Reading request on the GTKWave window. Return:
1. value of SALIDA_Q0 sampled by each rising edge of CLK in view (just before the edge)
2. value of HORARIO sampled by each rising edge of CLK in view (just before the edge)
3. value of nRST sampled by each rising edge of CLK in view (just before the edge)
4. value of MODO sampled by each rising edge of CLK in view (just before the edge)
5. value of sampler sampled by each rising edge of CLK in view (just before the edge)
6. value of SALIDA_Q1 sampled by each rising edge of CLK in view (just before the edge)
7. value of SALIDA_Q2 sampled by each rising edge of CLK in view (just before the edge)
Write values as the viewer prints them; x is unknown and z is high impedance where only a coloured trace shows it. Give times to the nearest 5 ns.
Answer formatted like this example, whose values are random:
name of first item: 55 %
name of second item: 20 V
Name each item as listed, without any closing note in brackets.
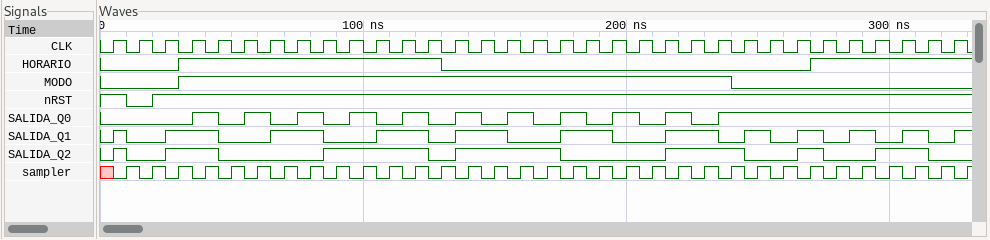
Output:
value of SALIDA_Q0 sampled by each rising edge of CLK in view: 0 0 0 0 1 0 1 0 1 0 1 0 1 0 1 0 1 0 1 0 1 0 1 0 1 1 1 1 1 1 1 1 1
value of HORARIO sampled by each rising edge of CLK in view: 0 0 0 1 1 1 1 1 1 1 1 1 1 0 0 0 0 0 0 0 0 0 0 0 0 0 0 1 1 1 1 1 1
value of nRST sampled by each rising edge of CLK in view: 1 0 1 1 1 1 1 1 1 1 1 1 1 1 1 1 1 1 1 1 1 1 1 1 1 1 1 1 1 1 1 1 1
value of MODO sampled by each rising edge of CLK in view: 0 0 0 1 1 1 1 1 1 1 1 1 1 1 1 1 1 1 1 1 1 1 1 1 0 0 0 0 0 0 0 0 0
value of sampler sampled by each rising edge of CLK in view: x 1 1 1 1 1 1 1 1 1 1 1 1 1 1 1 1 1 1 1 1 1 1 1 1 1 1 1 1 1 1 1 1
value of SALIDA_Q1 sampled by each rising edge of CLK in view: 0 0 0 1 1 0 0 1 1 0 0 1 1 0 1 1 0 0 1 1 0 0 1 1 0 1 0 1 0 1 0 1 0
value of SALIDA_Q2 sampled by each rising edge of CLK in view: 0 0 0 1 1 0 0 0 0 1 1 1 1 0 1 1 1 1 0 0 0 0 1 1 1 0 0 1 0 0 1 1 0
